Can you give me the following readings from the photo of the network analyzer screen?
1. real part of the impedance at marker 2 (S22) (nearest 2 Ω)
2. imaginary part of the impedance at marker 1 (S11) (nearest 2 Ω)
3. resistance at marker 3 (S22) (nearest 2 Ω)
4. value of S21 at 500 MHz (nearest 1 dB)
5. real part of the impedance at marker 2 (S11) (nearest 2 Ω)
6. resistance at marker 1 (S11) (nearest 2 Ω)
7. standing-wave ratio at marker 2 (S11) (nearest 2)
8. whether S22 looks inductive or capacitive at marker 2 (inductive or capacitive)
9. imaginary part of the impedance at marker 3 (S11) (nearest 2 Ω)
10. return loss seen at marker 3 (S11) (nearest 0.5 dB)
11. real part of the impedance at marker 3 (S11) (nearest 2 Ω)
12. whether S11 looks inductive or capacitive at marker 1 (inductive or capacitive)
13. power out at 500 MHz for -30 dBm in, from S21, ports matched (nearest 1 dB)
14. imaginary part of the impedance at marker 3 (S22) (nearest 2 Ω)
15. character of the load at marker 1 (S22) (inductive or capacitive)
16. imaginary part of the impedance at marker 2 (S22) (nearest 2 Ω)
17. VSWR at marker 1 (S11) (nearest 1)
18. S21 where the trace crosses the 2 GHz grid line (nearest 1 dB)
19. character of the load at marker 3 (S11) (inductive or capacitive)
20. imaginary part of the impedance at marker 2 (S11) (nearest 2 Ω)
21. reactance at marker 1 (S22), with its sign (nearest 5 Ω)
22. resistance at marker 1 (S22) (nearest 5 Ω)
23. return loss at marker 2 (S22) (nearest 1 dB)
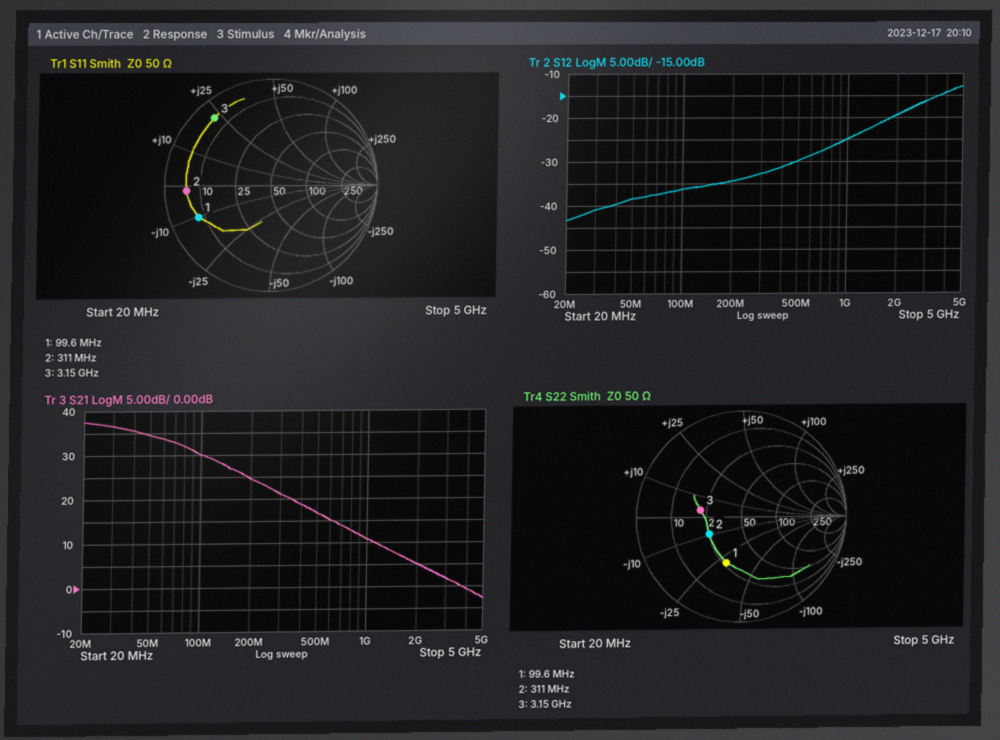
26 Ω
-10 Ω
22 Ω
17 dB
6 Ω
8 Ω
8
capacitive
+22 Ω
1.5 dB
6 Ω
capacitive
-13 dBm
+4 Ω
capacitive
-10 Ω
7
5 dB
inductive
-2 Ω
-30 Ω
25 Ω
9 dB
